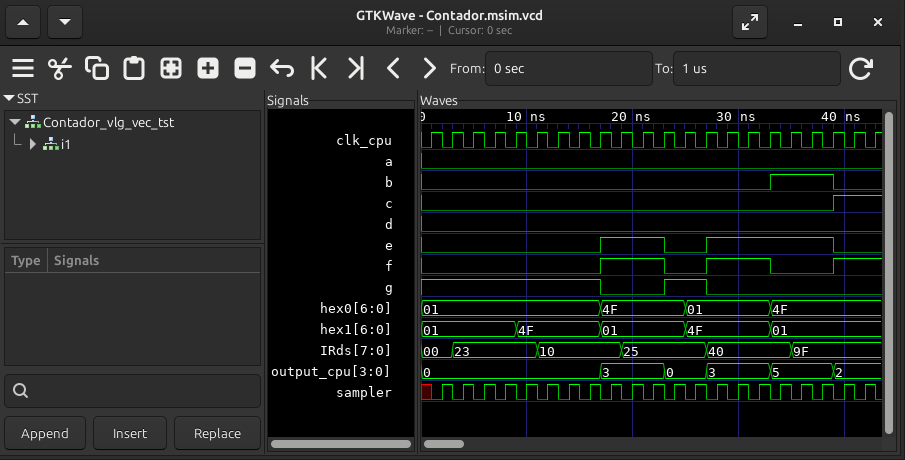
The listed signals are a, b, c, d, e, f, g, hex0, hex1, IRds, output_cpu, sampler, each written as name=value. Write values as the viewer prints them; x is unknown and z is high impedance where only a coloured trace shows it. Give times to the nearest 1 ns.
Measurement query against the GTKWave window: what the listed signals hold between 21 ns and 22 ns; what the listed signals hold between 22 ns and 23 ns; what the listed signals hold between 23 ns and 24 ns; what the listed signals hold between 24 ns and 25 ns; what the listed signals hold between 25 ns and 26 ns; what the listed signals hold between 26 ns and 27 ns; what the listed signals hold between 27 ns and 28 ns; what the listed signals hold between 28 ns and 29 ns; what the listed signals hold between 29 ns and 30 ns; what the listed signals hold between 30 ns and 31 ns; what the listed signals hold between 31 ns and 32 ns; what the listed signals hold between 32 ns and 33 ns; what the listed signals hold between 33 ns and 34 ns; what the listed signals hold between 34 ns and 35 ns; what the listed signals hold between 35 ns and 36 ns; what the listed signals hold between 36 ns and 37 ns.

a=0, b=0, c=0, d=0, e=1, f=1, g=0, hex0=4F, hex1=01, IRds=25, output_cpu=3, sampler=0
a=0, b=0, c=0, d=0, e=1, f=1, g=0, hex0=4F, hex1=01, IRds=25, output_cpu=3, sampler=1
a=0, b=0, c=0, d=0, e=0, f=0, g=1, hex0=4F, hex1=01, IRds=25, output_cpu=0, sampler=0
a=0, b=0, c=0, d=0, e=0, f=0, g=1, hex0=4F, hex1=01, IRds=25, output_cpu=0, sampler=1
a=0, b=0, c=0, d=0, e=0, f=0, g=1, hex0=01, hex1=4F, IRds=25, output_cpu=0, sampler=0
a=0, b=0, c=0, d=0, e=0, f=0, g=1, hex0=01, hex1=4F, IRds=25, output_cpu=0, sampler=1
a=0, b=0, c=0, d=0, e=1, f=1, g=0, hex0=01, hex1=4F, IRds=40, output_cpu=3, sampler=0
a=0, b=0, c=0, d=0, e=1, f=1, g=0, hex0=01, hex1=4F, IRds=40, output_cpu=3, sampler=1
a=0, b=0, c=0, d=0, e=1, f=1, g=0, hex0=01, hex1=4F, IRds=40, output_cpu=3, sampler=0
a=0, b=0, c=0, d=0, e=1, f=1, g=0, hex0=01, hex1=4F, IRds=40, output_cpu=3, sampler=1
a=0, b=0, c=0, d=0, e=1, f=1, g=0, hex0=01, hex1=4F, IRds=40, output_cpu=3, sampler=0
a=0, b=0, c=0, d=0, e=1, f=1, g=0, hex0=01, hex1=4F, IRds=40, output_cpu=3, sampler=1
a=0, b=1, c=0, d=0, e=1, f=0, g=0, hex0=4F, hex1=01, IRds=40, output_cpu=5, sampler=0
a=0, b=1, c=0, d=0, e=1, f=0, g=0, hex0=4F, hex1=01, IRds=40, output_cpu=5, sampler=1
a=0, b=1, c=0, d=0, e=1, f=0, g=0, hex0=4F, hex1=01, IRds=9F, output_cpu=5, sampler=0
a=0, b=1, c=0, d=0, e=1, f=0, g=0, hex0=4F, hex1=01, IRds=9F, output_cpu=5, sampler=1
